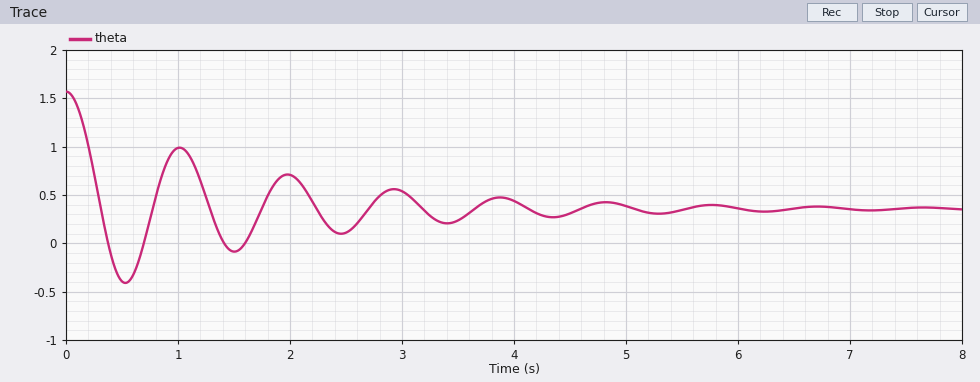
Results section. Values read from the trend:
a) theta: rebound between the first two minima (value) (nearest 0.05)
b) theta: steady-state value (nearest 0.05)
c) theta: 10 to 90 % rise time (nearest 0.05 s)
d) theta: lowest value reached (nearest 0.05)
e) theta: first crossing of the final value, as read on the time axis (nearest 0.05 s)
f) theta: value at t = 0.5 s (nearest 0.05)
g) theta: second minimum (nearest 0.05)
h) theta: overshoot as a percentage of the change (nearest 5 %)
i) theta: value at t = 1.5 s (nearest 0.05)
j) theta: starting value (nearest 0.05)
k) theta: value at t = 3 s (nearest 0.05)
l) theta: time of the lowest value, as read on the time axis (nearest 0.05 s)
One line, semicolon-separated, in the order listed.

1.00; 0.35; 0.20 s; -0.40; 0.30 s; -0.40; -0.10; 65 %; -0.10; 1.55; 0.55; 0.55 s
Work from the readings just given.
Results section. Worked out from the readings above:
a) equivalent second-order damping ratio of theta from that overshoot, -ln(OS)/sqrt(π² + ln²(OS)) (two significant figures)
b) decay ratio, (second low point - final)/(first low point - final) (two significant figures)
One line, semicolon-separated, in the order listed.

0.14; 0.60
